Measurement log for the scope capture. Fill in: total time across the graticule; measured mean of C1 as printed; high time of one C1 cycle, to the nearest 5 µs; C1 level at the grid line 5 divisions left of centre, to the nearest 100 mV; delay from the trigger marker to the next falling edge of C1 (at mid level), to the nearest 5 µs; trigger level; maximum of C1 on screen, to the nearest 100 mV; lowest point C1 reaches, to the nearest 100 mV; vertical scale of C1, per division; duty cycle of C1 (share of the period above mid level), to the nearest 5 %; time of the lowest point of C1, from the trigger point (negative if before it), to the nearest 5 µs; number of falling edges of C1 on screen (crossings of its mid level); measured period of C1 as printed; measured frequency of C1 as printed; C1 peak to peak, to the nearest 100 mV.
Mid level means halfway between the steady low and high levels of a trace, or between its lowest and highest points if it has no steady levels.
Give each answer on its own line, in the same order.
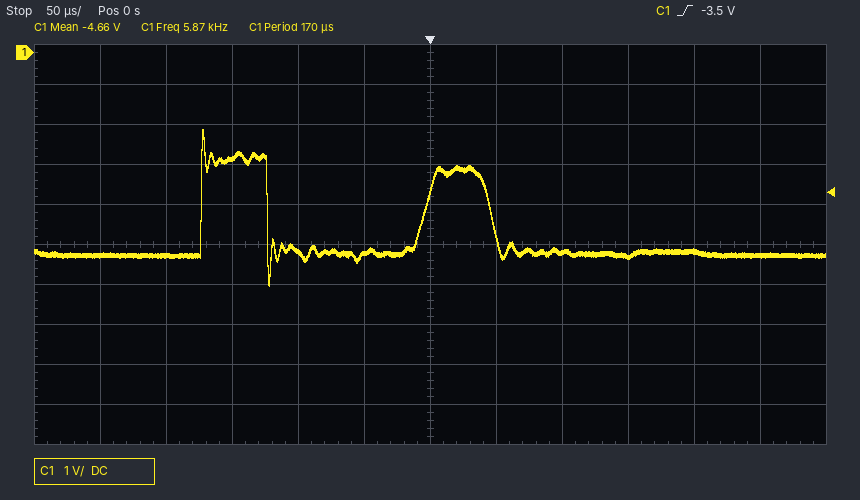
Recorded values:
600 µs
-4.66 V
50 µs
-5.1 V
45 µs
-3.5 V
-1.9 V
-5.8 V
1 V
30 %
-120 µs
2
170 µs
5.87 kHz
3.9 V
